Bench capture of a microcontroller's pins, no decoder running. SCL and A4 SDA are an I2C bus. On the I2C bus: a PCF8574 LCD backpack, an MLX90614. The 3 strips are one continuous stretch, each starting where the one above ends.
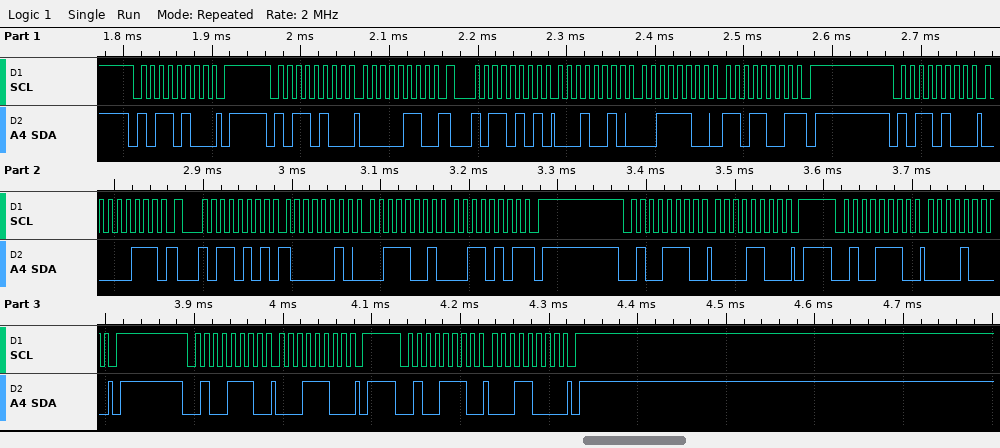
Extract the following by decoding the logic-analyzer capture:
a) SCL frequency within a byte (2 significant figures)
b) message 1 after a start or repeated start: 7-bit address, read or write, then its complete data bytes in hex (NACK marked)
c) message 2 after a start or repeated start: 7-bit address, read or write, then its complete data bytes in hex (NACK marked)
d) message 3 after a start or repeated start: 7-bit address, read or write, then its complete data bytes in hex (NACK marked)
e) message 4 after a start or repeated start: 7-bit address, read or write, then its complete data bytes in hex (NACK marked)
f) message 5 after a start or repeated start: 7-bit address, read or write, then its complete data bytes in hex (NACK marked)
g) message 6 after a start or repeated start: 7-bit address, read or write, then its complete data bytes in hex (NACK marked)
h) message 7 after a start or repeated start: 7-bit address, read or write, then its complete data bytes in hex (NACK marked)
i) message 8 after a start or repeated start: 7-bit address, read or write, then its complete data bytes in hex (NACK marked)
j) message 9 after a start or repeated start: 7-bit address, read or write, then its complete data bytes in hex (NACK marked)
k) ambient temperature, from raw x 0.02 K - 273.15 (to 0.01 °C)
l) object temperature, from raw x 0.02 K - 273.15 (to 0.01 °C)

100 kHz
0x5A write
0x5A write: 06
0x5A read: 12 3C D9 NACK
0x5A write: 07
0x5A read: 82 39 35 NACK
0x27 write: 0C
0x27 write: 08
0x27 write: 1C
0x27 write: 18
34.41 °C
21.29 °C
